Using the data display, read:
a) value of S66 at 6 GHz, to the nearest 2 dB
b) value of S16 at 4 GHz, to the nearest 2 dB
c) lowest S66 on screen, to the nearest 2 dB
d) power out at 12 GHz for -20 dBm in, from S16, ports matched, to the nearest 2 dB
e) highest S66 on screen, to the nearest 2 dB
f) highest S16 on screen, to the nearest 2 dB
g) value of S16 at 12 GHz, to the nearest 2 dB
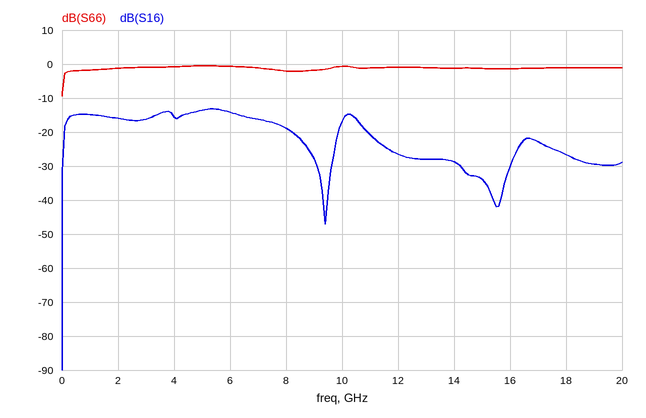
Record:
0 dB
-16 dB
-10 dB
-46 dBm
0 dB
-14 dB
-26 dB
